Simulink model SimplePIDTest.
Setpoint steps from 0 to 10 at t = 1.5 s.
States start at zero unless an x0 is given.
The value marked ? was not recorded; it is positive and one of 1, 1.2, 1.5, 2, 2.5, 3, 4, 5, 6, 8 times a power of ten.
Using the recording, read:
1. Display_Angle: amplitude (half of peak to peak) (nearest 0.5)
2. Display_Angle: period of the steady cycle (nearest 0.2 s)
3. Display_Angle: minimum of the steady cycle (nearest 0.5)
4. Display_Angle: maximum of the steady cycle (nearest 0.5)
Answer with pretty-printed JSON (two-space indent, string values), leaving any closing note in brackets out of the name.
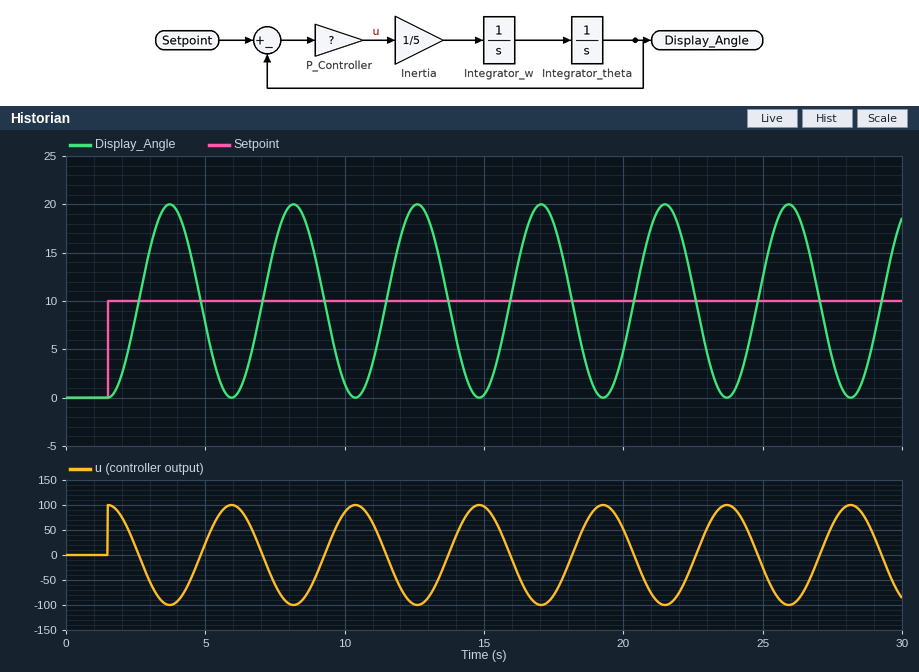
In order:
{
  "Display_Angle: amplitude (half of peak to peak)": "10.0",
  "Display_Angle: period of the steady cycle": "4.4 s",
  "Display_Angle: minimum of the steady cycle": "0.0",
  "Display_Angle: maximum of the steady cycle": "20.0"
}
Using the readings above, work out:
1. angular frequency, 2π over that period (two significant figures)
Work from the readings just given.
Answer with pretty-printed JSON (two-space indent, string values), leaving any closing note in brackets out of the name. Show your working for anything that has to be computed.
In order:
{
  "angular frequency, 2π over that period": "2π / 4.4 = 1.4 rad/s"
}
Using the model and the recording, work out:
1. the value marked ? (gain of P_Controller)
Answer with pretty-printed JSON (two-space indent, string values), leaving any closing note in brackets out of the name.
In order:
{
  "the value marked ?": "10"
}
